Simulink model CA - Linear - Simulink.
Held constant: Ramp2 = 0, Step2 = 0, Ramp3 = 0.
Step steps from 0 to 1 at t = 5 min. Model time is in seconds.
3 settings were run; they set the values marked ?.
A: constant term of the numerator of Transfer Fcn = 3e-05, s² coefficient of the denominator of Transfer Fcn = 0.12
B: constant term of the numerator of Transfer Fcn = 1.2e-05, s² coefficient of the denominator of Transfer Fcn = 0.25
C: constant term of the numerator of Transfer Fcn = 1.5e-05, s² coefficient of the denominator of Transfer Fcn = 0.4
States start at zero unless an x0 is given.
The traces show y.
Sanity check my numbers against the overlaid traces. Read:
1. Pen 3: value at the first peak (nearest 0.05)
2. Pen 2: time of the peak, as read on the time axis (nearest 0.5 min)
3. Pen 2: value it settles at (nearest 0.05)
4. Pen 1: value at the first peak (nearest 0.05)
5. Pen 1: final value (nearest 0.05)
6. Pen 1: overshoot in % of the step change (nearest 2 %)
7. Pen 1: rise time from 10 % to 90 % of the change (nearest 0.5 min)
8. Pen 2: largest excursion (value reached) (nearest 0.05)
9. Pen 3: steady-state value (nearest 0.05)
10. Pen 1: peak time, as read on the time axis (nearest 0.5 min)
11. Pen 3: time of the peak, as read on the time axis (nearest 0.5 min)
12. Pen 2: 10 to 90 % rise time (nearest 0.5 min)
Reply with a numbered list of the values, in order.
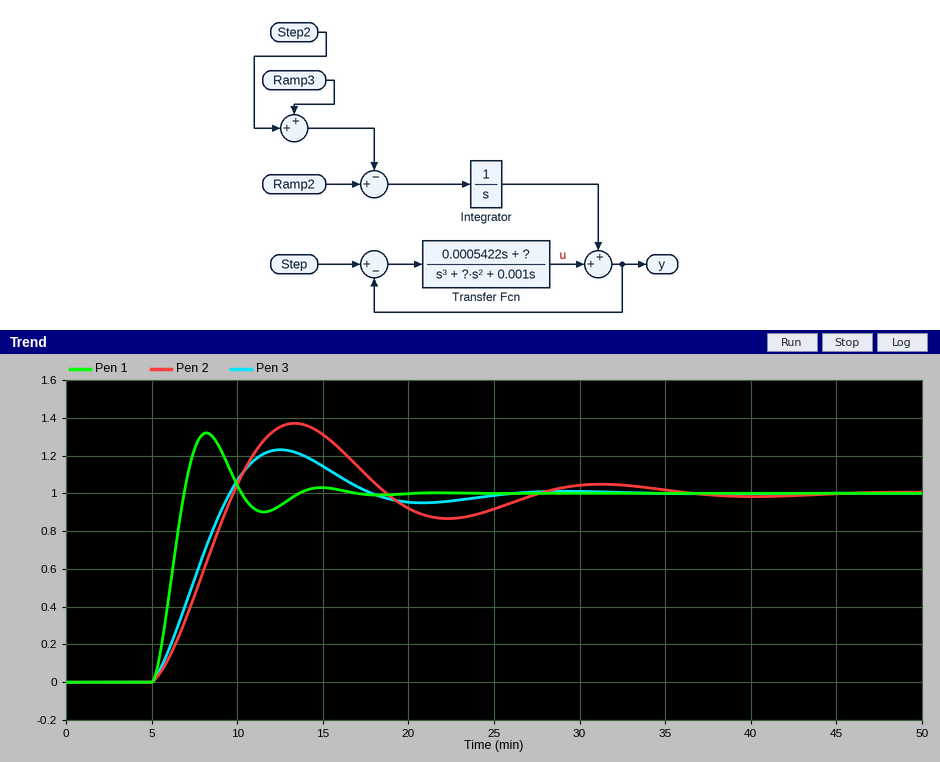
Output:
1. 1.25
2. 13.5 min
3. 1.00
4. 1.30
5. 1.00
6. 32 %
7. 1.5 min
8. 1.35
9. 1.00
10. 8.0 min
11. 12.5 min
12. 3.5 min
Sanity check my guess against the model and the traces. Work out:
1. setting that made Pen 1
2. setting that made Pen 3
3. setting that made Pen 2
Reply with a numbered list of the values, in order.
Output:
1. A
2. B
3. C
